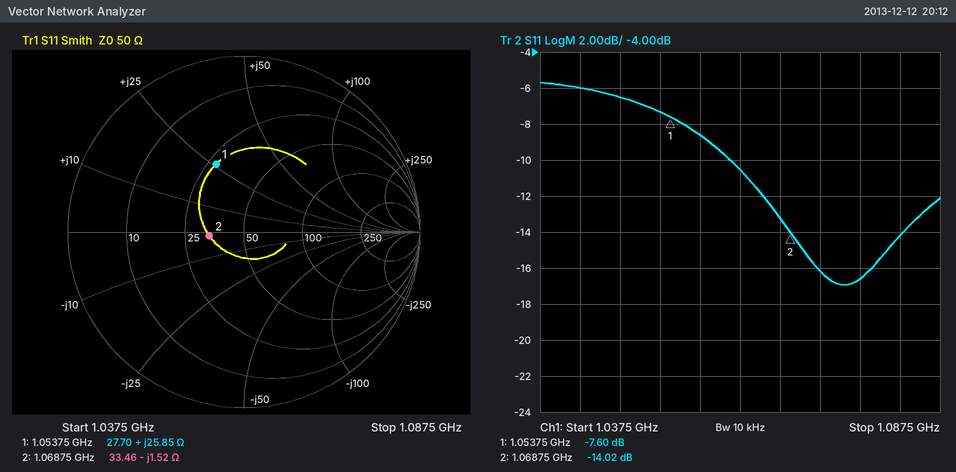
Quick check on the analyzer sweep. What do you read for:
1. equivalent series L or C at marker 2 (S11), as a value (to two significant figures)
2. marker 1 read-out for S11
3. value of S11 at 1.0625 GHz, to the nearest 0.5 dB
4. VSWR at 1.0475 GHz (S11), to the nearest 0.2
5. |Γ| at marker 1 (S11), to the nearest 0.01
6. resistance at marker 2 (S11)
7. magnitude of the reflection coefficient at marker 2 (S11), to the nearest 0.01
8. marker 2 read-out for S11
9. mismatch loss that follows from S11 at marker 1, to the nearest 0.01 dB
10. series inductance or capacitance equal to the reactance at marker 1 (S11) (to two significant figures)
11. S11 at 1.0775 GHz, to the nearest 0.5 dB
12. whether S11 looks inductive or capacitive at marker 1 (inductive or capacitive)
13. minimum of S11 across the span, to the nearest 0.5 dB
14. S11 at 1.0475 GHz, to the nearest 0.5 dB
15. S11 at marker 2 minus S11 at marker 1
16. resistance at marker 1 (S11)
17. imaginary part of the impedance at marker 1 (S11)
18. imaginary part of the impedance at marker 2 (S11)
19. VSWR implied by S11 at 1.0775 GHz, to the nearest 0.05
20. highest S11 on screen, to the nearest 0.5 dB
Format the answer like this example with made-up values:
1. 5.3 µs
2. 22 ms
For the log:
1. 98 pF
2. -7.60 dB
3. -10.5 dB
4. 2.8
5. 0.42
6. 33.46 Ω
7. 0.20
8. -14.02 dB
9. 0.83 dB
10. 3.9 nH
11. -16.5 dB
12. inductive
13. -17.0 dB
14. -6.5 dB
15. -6.42 dB
16. 27.70 Ω
17. +25.85 Ω
18. -1.52 Ω
19. 1.35
20. -5.5 dB
